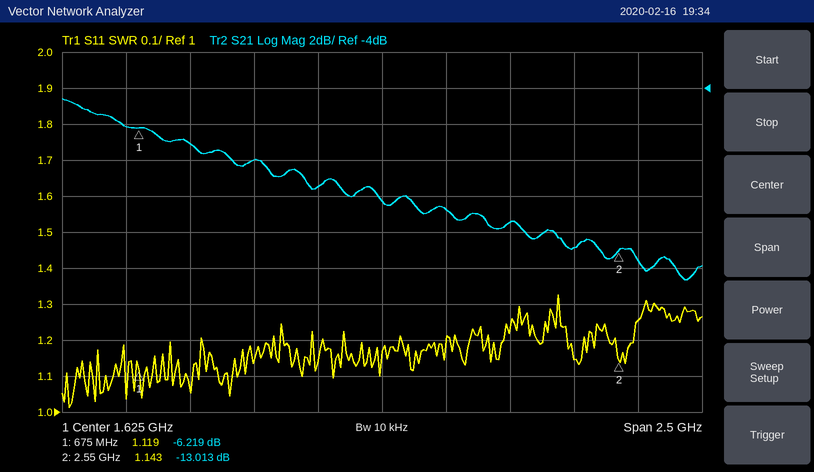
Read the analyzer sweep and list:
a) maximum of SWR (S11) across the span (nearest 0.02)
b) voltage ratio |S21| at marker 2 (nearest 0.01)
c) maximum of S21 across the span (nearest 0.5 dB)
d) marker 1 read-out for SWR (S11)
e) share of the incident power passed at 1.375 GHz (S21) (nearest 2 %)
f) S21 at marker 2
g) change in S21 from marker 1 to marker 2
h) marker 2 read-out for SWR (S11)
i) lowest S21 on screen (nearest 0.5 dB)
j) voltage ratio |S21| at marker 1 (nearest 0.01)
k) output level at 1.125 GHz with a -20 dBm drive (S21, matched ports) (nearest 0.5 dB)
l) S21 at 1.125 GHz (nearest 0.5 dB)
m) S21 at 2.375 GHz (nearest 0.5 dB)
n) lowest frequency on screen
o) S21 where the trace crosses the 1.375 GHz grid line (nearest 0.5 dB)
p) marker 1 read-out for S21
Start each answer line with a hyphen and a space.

- 1.32
- 0.22
- -4.5 dB
- 1.119
- 12 %
- -13.013 dB
- -6.794 dB
- 1.143
- -14.5 dB
- 0.49
- -28.0 dBm
- -8.0 dB
- -13.0 dB
- 375 MHz
- -9.5 dB
- -6.219 dB
